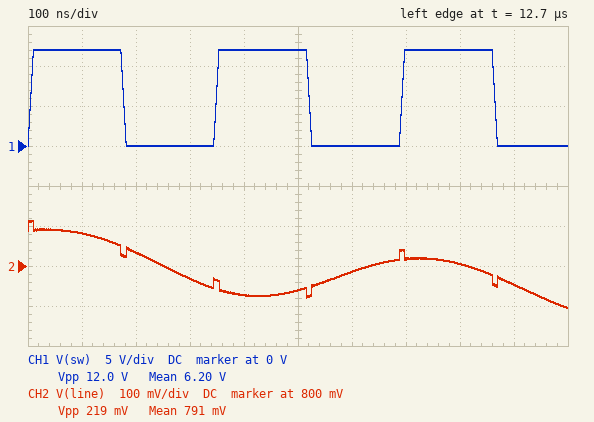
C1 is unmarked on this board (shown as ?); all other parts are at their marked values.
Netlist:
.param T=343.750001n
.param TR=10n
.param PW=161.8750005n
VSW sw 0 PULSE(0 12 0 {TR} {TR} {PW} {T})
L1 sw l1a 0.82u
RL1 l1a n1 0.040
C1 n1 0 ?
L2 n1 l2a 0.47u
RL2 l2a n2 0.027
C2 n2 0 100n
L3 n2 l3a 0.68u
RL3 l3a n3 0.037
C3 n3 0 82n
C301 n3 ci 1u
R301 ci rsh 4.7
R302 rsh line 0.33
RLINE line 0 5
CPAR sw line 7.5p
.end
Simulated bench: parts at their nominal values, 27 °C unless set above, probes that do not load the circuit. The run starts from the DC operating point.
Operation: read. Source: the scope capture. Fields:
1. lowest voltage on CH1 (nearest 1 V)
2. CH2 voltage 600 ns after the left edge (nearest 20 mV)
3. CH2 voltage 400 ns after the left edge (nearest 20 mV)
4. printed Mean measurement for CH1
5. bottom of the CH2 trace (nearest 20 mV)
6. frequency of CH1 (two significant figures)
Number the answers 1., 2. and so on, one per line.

1. 0 V
2. 780 mV
3. 720 mV
4. 6.20 V
5. 700 mV
6. 2.9 MHz
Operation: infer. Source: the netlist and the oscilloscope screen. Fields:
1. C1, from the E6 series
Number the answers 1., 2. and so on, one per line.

1. 47 nF
